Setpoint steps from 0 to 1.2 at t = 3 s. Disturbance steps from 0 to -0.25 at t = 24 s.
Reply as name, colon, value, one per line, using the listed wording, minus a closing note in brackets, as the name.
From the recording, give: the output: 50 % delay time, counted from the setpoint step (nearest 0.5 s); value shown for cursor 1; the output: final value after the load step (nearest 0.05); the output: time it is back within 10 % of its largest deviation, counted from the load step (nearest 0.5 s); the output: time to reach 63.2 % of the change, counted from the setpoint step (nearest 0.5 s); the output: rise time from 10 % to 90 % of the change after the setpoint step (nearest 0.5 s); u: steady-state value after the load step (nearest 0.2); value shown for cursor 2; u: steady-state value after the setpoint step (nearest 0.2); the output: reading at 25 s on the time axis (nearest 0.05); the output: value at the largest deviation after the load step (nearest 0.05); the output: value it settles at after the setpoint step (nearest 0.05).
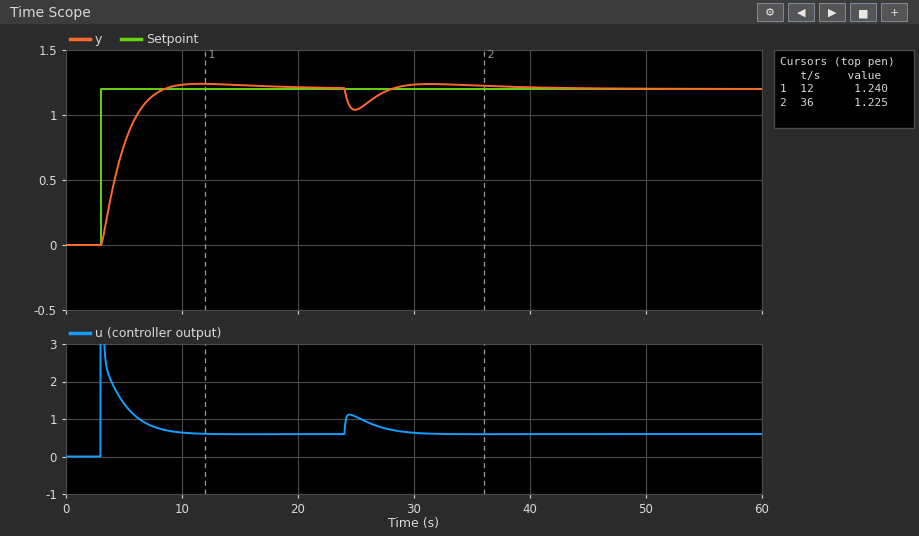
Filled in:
the output: 50 % delay time, counted from the setpoint step: 1.5 s
value shown for cursor 1: 1.240
the output: final value after the load step: 1.20
the output: time it is back within 10 % of its largest deviation, counted from the load step: 14.5 s
the output: time to reach 63.2 % of the change, counted from the setpoint step: 2.0 s
the output: rise time from 10 % to 90 % of the change after the setpoint step: 3.5 s
u: steady-state value after the load step: 0.6
value shown for cursor 2: 1.225
u: steady-state value after the setpoint step: 0.6
the output: reading at 25 s on the time axis: 1.05
the output: value at the largest deviation after the load step: 1.05
the output: value it settles at after the setpoint step: 1.20
